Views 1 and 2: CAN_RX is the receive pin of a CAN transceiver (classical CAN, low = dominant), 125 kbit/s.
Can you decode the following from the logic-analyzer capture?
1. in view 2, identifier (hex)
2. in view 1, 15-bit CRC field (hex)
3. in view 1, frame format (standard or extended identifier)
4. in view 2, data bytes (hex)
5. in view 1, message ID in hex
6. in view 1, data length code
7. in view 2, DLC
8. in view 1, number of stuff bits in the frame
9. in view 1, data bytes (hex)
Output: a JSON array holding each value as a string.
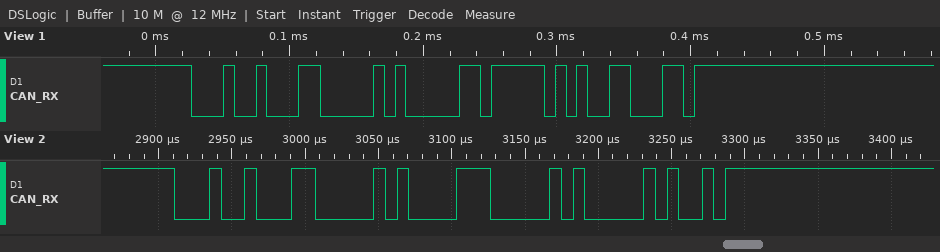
["0x123", "0x7D31", "standard", "0E", "0x123", "1", "1", "3", "05"]
